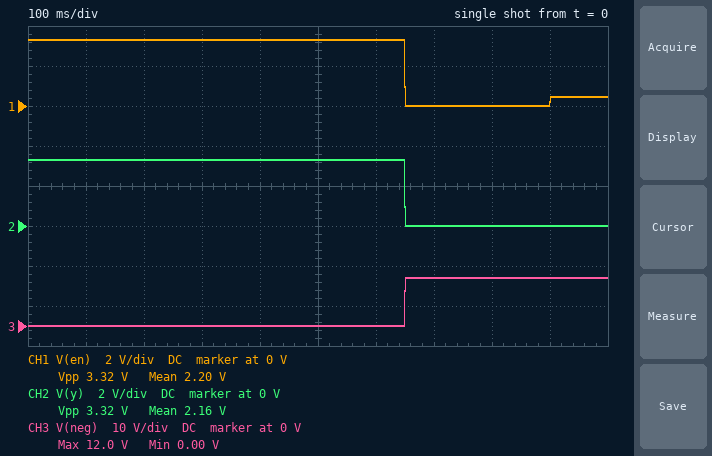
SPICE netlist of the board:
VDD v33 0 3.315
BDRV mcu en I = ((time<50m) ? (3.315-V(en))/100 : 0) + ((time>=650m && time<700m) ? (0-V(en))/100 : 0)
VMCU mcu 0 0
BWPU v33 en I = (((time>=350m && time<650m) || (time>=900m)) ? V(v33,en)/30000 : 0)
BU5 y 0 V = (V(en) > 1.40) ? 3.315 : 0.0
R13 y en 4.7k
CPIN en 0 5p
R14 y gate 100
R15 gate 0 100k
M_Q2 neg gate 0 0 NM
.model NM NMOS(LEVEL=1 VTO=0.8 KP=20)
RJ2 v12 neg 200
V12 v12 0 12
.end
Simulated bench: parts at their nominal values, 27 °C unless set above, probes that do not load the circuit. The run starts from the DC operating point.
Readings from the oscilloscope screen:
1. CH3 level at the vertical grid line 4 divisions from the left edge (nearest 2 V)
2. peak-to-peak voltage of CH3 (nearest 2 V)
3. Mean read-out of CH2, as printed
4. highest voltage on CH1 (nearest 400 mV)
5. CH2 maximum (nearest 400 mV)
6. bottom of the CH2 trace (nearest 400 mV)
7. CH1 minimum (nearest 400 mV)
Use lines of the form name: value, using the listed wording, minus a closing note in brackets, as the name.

CH3 level at the vertical grid line 4 divisions from the left edge: 0 V
peak-to-peak voltage of CH3: 12 V
Mean read-out of CH2, as printed: 2.16 V
highest voltage on CH1: 3.2 V
CH2 maximum: 3.2 V
bottom of the CH2 trace: 0 V
CH1 minimum: 0 V
